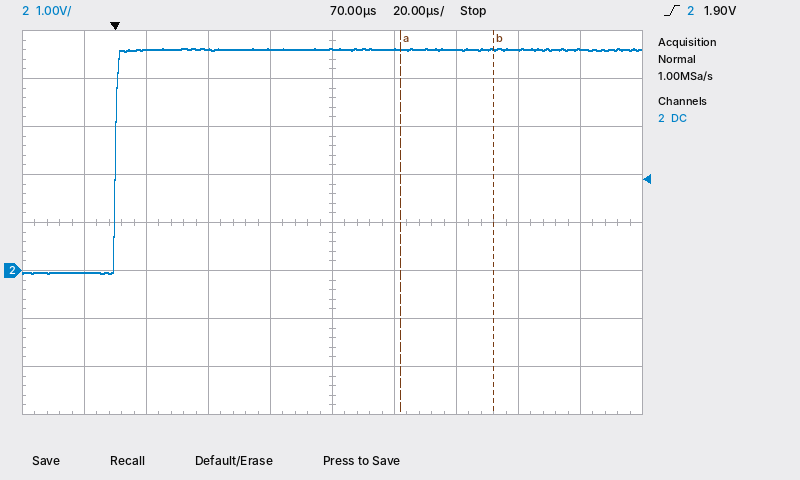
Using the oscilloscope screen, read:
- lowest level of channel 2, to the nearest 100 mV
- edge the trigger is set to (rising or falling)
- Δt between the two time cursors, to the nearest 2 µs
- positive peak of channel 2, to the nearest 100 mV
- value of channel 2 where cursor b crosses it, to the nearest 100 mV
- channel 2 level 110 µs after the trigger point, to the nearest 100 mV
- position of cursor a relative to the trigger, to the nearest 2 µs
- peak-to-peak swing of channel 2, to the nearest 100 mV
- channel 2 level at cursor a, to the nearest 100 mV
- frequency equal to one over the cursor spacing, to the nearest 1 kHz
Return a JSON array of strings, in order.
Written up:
["-100 mV", "rising", "30 µs", "4.6 V", "4.6 V", "4.6 V", "+92 µs", "4.7 V", "4.6 V", "33 kHz"]
